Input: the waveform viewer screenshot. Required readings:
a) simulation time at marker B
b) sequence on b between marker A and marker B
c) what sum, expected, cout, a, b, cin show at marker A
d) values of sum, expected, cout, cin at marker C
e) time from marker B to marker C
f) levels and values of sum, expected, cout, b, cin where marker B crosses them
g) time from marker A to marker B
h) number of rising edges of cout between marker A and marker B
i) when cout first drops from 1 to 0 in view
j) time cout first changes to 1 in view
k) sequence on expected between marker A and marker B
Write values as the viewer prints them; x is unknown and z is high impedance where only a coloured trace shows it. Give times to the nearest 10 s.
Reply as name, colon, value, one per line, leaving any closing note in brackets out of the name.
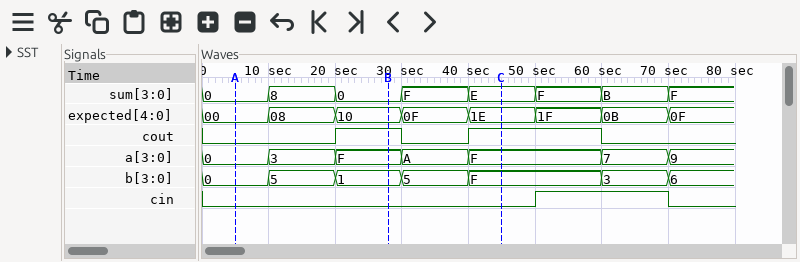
simulation time at marker B: 30 s
sequence on b between marker A and marker B: 0, 5, 1
what sum, expected, cout, a, b, cin show at marker A: sum=0, expected=00, cout=0, a=0, b=0, cin=0
values of sum, expected, cout, cin at marker C: sum=E, expected=1E, cout=1, cin=0
time from marker B to marker C: 20 s
levels and values of sum, expected, cout, b, cin where marker B crosses them: sum=0, expected=10, cout=1, b=1, cin=0
time from marker A to marker B: 20 s
number of rising edges of cout between marker A and marker B: 1
when cout first drops from 1 to 0 in view: 30 s
time cout first changes to 1 in view: 20 s
sequence on expected between marker A and marker B: 00, 08, 10
